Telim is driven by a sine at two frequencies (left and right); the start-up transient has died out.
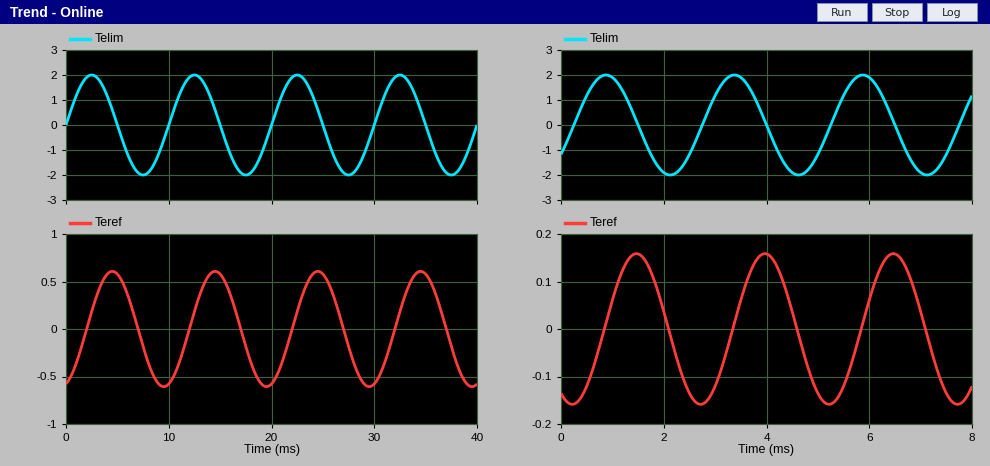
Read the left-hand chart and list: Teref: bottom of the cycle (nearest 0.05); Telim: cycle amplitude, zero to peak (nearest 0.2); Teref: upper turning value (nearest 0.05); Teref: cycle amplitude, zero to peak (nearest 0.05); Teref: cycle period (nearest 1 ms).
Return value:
-0.60
2.0
0.60
0.60
10 ms
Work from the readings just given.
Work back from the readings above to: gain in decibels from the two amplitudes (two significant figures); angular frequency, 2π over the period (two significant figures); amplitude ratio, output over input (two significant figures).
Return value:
-10 dB
0.63 rad/ms
0.30
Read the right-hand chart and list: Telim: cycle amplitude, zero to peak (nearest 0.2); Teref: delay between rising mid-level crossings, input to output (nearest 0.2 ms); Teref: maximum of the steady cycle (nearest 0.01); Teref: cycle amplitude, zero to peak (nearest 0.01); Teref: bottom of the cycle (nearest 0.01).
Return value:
2.0
0.6 ms
0.16
0.16
-0.16
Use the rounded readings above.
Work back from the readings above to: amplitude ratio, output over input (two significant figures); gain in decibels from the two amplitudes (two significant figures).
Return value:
0.080
-22 dB
